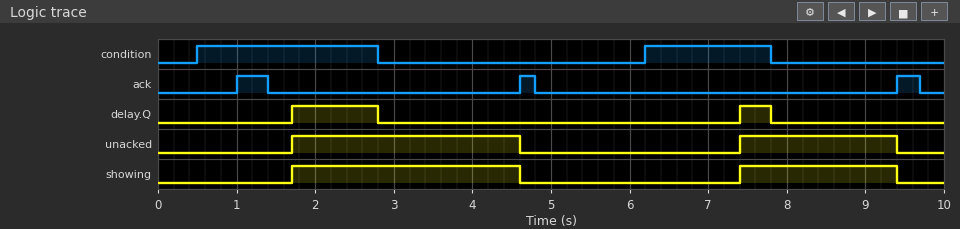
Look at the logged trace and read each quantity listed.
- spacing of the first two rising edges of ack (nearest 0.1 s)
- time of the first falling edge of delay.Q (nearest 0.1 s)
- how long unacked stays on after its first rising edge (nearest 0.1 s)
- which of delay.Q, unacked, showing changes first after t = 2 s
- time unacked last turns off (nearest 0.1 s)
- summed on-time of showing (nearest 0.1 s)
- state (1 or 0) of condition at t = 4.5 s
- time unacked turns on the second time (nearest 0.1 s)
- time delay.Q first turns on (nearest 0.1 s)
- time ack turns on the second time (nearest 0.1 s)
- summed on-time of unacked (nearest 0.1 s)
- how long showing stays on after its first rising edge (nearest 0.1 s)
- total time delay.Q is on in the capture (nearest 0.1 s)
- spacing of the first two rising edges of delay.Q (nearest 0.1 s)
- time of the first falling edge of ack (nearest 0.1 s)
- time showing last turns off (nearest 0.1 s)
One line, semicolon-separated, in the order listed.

3.6 s; 2.8 s; 2.9 s; delay.Q; 9.4 s; 4.9 s; 0; 7.4 s; 1.7 s; 4.6 s; 4.9 s; 2.9 s; 1.5 s; 5.7 s; 1.4 s; 9.4 s
